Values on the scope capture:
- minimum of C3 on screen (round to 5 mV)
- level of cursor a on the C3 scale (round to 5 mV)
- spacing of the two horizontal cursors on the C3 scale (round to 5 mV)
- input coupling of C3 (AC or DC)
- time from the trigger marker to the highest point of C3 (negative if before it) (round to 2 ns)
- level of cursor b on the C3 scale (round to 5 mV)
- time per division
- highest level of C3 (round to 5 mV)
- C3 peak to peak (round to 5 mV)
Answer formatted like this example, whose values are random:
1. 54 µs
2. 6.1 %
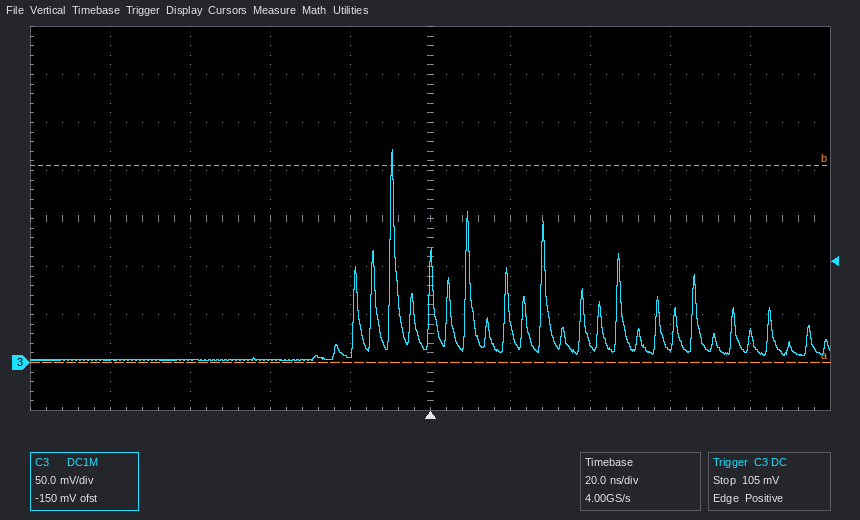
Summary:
1. 0 mV
2. 0 mV
3. 205 mV
4. DC
5. -10 ns
6. 205 mV
7. 20 ns
8. 220 mV
9. 220 mV
